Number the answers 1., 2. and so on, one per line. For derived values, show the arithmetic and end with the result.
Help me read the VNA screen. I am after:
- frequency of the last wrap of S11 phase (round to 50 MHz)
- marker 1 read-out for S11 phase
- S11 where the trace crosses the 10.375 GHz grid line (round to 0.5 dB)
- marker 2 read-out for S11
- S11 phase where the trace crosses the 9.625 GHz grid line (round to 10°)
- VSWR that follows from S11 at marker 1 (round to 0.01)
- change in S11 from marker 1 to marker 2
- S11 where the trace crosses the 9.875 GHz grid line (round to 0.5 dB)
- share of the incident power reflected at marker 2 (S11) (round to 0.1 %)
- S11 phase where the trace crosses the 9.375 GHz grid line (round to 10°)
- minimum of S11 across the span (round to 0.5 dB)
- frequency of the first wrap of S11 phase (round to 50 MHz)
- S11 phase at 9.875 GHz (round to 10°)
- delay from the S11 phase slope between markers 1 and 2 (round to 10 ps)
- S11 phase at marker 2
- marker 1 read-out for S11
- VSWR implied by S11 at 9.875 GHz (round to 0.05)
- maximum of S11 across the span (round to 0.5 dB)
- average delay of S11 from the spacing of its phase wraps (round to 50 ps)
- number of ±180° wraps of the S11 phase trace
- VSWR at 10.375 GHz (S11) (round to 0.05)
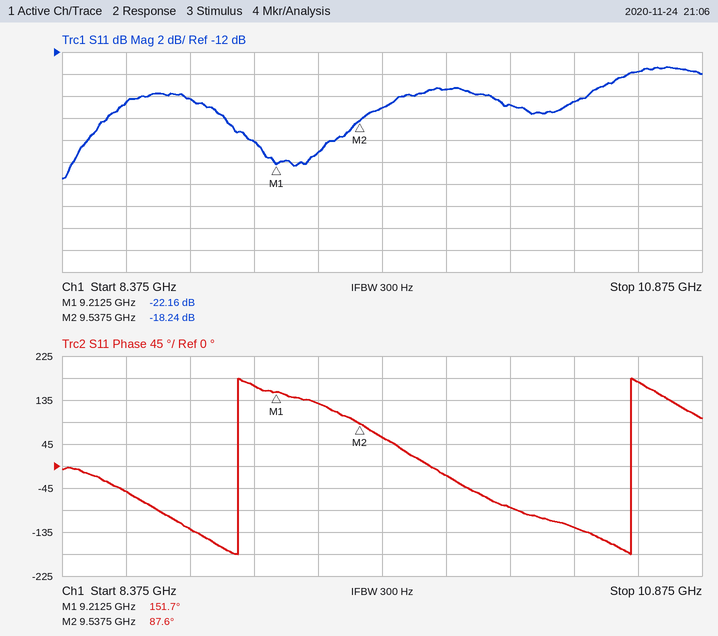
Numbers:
1. 10.60 GHz
2. 151.7°
3. -16.5 dB
4. -18.24 dB
5. 60°
6. (1 + 0.0780)/(1 − 0.0780) ≈ 1.17
7. -18.24 − (-22.16) = 3.92 dB
8. -15.5 dB
9. 10^(-18.24/10) ≈ 1.5 %
10. 130°
11. -23.5 dB
12. 9.05 GHz
13. -20°
14. −(87.6° − (151.7°))/(360° × 325 MHz) ≈ 548 ps, so 550 ps to the nearest 10 ps
15. 87.6°
16. -22.16 dB
17. |Γ| = 10^(-15.5/20) = 0.1679; VSWR = (1 + 0.1679)/(1 − 0.1679) ≈ 1.40
18. -13.5 dB
19. 1 cycle / (10.60 GHz − 9.05 GHz) ≈ 645 ps, so 650 ps to the nearest 50 ps
20. 2
21. |Γ| = 10^(-16.5/20) = 0.1496; VSWR = (1 + 0.1496)/(1 − 0.1496) ≈ 1.35
